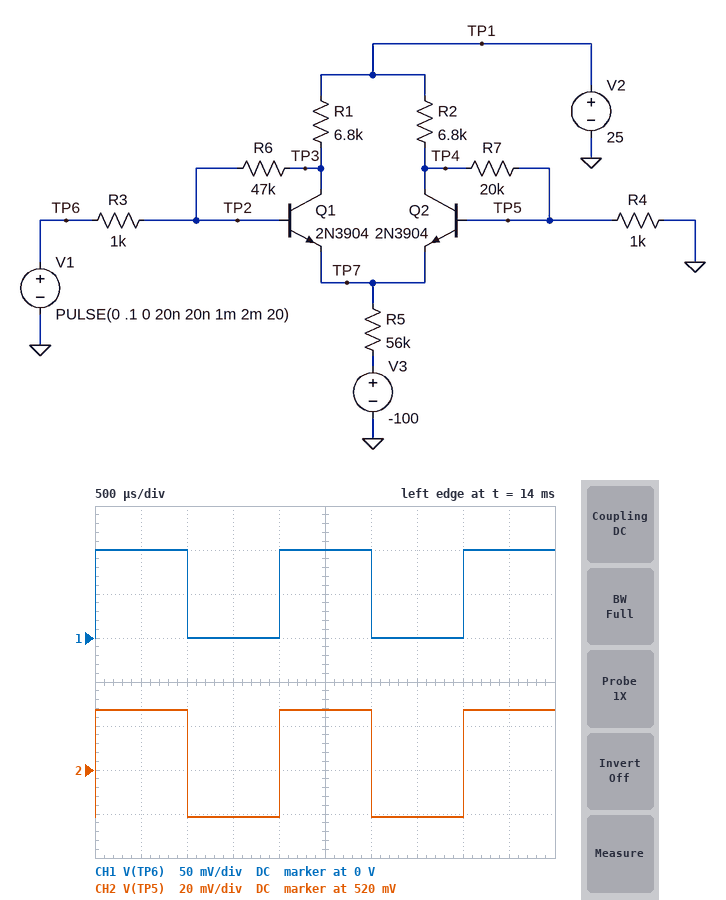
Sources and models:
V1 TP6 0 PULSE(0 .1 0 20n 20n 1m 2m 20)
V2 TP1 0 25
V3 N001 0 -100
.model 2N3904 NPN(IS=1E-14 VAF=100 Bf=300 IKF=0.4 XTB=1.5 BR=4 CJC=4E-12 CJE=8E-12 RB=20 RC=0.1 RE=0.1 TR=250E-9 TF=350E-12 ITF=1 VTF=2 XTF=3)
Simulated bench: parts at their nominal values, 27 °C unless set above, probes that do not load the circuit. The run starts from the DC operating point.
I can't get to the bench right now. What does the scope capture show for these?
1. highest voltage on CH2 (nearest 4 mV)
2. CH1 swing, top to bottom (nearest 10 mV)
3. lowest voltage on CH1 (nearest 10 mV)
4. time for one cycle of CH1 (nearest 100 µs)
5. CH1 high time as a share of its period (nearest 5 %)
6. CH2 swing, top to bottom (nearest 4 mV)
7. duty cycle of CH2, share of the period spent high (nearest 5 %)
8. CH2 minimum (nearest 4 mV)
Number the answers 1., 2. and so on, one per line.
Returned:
1. 548 mV
2. 100 mV
3. 0 V
4. 2.0 ms
5. 50 %
6. 48 mV
7. 50 %
8. 500 mV
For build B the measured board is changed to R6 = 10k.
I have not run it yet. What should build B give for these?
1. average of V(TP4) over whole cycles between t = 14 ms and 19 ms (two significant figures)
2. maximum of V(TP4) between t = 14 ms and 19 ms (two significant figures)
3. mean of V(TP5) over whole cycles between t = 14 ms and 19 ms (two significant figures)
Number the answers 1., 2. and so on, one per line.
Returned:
1. 17 V
2. 18 V
3. 830 mV
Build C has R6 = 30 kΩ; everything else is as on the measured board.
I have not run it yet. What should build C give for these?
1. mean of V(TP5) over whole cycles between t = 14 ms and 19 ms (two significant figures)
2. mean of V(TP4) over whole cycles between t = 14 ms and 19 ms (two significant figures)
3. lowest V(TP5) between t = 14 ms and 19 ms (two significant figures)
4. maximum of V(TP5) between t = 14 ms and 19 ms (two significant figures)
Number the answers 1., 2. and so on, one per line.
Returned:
1. 610 mV
2. 13 V
3. 590 mV
4. 640 mV
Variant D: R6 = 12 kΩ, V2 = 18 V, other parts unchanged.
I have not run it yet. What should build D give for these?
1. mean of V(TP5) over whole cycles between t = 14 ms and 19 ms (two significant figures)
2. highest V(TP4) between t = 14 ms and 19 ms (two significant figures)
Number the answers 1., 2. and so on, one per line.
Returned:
1. 510 mV
2. 11 V
